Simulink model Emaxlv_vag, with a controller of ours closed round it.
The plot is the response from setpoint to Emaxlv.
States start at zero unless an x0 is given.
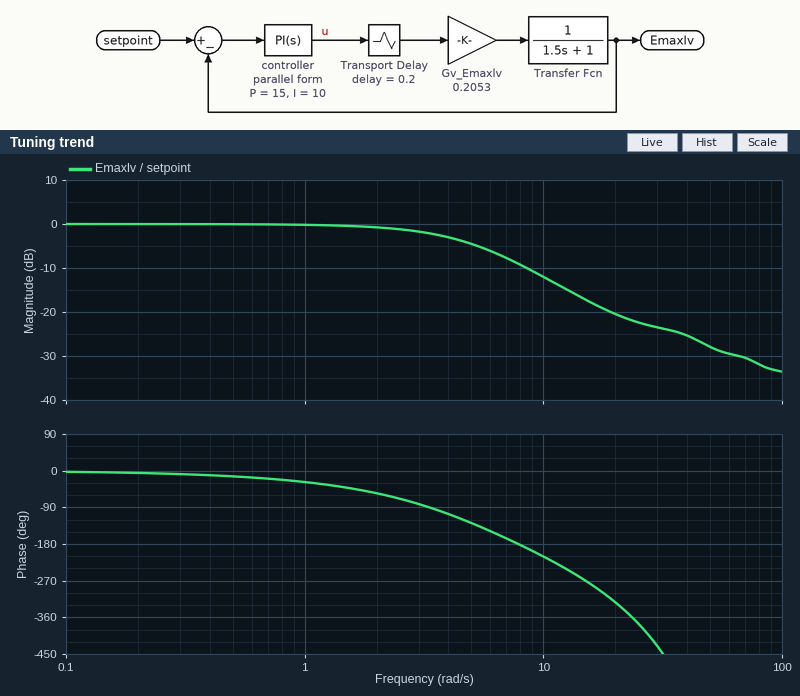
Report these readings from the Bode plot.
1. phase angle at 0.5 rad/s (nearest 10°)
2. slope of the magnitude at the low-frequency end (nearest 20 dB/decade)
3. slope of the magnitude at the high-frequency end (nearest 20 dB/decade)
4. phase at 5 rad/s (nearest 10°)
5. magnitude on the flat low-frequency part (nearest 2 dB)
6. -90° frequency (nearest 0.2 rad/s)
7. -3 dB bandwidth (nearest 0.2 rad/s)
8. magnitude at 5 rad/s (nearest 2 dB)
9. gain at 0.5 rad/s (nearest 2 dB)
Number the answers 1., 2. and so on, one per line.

1. -10°
2. 0 dB/decade
3. -20 dB/decade
4. -130°
5. 0 dB
6. 3.4 rad/s
7. 4.0 rad/s
8. -4 dB
9. 0 dB
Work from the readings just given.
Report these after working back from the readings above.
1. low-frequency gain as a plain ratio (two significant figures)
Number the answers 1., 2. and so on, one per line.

1. 1.0
